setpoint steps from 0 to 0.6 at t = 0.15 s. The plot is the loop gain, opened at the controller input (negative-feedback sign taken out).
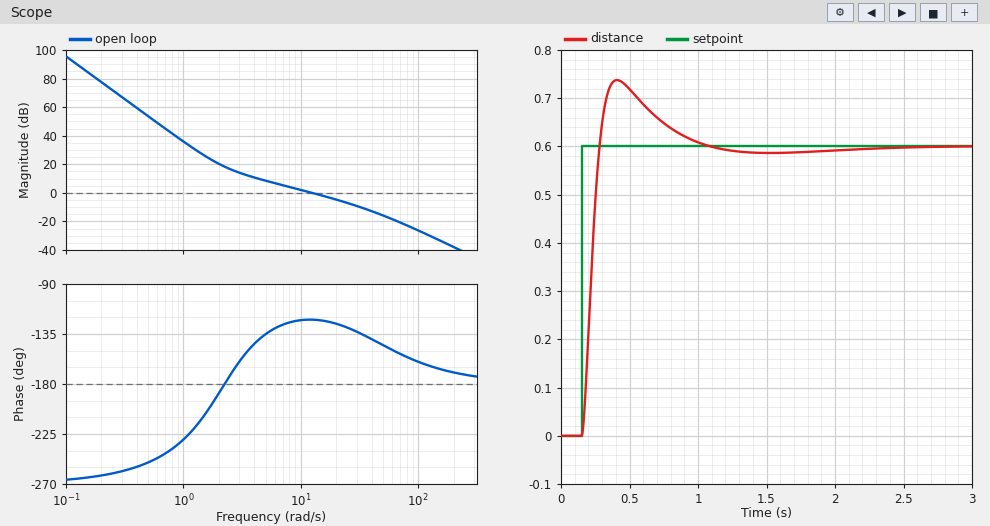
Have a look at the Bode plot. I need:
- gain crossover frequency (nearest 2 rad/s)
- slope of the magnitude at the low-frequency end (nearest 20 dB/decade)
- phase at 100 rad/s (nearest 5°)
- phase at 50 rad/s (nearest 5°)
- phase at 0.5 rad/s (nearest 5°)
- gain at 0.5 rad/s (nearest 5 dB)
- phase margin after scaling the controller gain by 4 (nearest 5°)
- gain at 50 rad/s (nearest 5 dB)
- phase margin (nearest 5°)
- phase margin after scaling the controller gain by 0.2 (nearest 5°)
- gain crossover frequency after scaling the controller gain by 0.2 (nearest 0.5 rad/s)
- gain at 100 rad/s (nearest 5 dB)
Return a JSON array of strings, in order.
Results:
["12 rad/s", "-60 dB/decade", "-160°", "-145°", "-250°", "55 dB", "40°", "-15 dB", "60°", "20°", "3.0 rad/s", "-25 dB"]
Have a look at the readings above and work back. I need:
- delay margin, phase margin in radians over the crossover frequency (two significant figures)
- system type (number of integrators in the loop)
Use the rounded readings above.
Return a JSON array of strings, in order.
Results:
["0.087 s", "3"]
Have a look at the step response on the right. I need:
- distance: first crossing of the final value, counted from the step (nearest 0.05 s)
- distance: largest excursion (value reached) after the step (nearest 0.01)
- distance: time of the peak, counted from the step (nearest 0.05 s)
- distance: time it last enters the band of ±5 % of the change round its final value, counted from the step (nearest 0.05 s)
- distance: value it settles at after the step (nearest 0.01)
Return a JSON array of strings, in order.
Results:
["0.15 s", "0.74", "0.25 s", "0.70 s", "0.60"]
